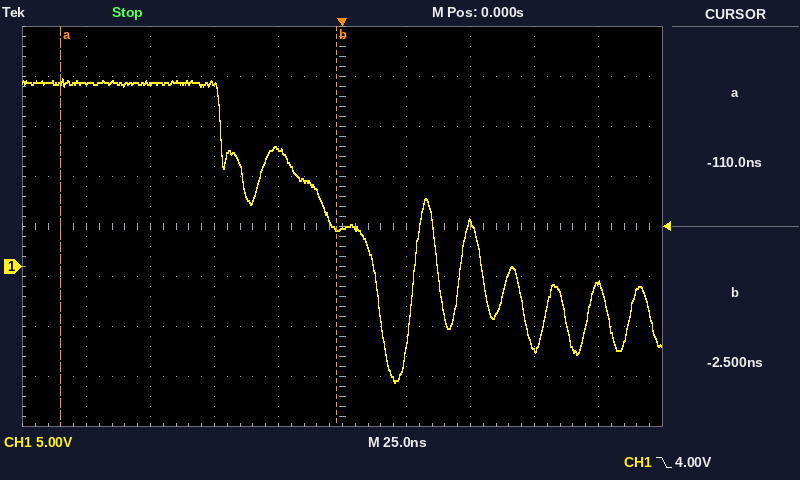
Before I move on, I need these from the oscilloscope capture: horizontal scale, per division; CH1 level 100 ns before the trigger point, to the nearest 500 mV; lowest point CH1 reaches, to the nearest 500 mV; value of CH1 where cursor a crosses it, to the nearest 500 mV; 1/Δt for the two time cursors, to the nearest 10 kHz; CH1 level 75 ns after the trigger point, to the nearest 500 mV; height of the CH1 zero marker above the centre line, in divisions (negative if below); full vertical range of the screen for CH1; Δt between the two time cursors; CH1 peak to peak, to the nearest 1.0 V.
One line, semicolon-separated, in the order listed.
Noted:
25 ns; 18.5 V; -11.5 V; 18.5 V; 9.30 MHz; -8.0 V; -0.8 div; 40 V; 107.5 ns; 30.0 V
